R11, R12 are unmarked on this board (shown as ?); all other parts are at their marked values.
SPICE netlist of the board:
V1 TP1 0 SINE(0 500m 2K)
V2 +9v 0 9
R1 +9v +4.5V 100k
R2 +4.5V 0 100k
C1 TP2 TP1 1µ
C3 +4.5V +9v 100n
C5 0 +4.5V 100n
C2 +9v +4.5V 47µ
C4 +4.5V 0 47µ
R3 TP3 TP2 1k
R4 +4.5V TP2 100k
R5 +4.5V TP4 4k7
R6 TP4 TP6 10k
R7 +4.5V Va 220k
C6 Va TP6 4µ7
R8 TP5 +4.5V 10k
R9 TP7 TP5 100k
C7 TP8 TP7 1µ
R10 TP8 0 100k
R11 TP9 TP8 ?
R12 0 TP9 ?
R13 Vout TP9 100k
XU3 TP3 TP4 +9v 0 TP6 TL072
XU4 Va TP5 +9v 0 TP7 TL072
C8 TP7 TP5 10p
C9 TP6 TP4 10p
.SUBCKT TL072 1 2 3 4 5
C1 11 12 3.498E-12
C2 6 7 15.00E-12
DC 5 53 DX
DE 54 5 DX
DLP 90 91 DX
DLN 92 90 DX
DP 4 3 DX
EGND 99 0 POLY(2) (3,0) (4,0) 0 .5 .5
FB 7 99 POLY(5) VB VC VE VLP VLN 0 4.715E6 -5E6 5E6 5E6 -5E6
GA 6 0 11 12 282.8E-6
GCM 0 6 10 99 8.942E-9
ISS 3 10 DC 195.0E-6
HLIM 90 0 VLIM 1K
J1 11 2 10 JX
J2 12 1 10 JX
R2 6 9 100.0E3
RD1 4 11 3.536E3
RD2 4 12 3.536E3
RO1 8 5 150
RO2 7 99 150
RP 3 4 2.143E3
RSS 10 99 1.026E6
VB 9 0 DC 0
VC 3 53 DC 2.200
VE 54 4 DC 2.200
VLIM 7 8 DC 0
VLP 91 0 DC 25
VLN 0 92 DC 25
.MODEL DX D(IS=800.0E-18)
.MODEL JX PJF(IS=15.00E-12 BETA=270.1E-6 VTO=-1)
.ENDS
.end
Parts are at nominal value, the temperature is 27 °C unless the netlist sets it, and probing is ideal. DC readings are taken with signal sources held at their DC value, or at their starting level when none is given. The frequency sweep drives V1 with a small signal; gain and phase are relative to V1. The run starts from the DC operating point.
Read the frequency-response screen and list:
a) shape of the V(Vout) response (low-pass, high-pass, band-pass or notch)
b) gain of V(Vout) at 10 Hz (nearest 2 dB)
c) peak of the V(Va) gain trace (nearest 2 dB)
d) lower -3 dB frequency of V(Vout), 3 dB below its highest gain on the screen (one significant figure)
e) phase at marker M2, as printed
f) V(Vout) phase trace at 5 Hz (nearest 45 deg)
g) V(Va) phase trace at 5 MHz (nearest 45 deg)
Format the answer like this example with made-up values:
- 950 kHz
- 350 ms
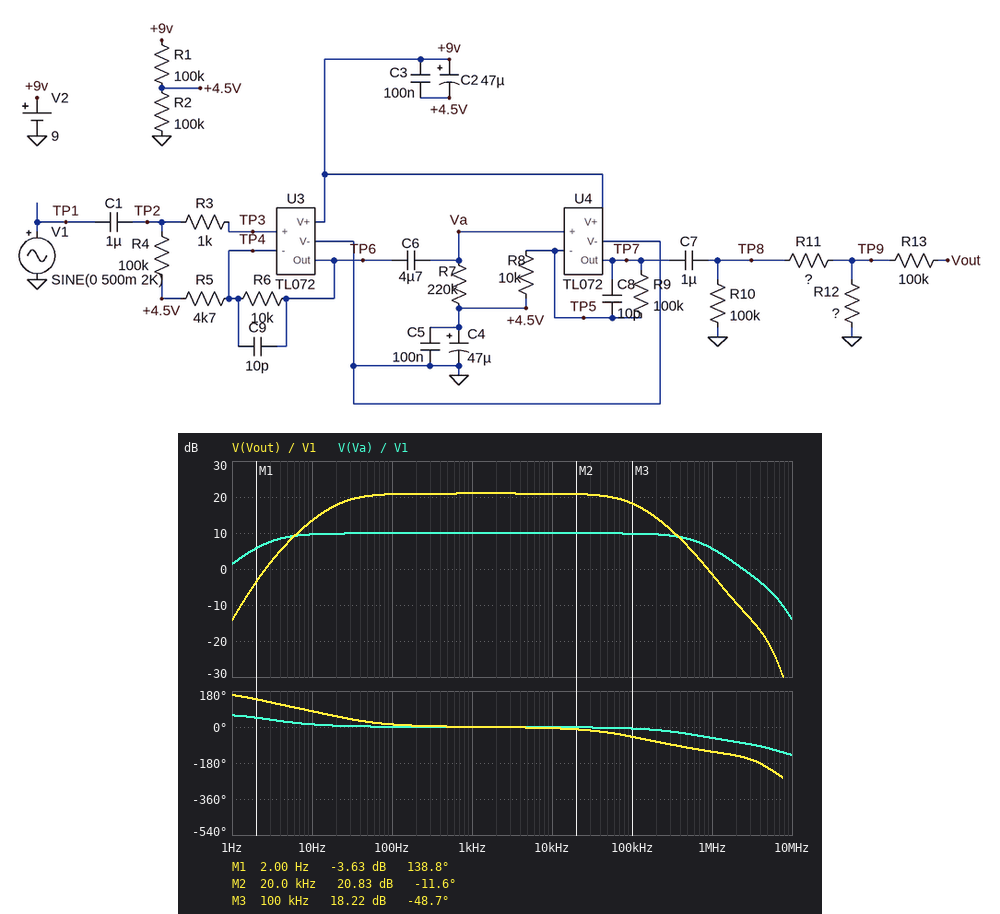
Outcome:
- band-pass
- 14 dB
- 10 dB
- 20 Hz
- -11.6 deg
- 90 deg
- -90 deg
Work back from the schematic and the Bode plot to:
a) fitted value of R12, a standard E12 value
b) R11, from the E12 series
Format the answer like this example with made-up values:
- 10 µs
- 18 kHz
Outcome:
- 2.7 kΩ
- 5.6 kΩ
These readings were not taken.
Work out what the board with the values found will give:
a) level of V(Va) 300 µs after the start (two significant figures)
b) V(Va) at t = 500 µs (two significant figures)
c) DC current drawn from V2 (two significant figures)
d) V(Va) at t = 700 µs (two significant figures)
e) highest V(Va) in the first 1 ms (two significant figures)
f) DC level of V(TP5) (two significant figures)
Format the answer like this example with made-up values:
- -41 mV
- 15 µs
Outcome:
- 3.6 V
- 4.5 V
- 8.8 mA
- 5.4 V
- 6.1 V
- 4.5 V
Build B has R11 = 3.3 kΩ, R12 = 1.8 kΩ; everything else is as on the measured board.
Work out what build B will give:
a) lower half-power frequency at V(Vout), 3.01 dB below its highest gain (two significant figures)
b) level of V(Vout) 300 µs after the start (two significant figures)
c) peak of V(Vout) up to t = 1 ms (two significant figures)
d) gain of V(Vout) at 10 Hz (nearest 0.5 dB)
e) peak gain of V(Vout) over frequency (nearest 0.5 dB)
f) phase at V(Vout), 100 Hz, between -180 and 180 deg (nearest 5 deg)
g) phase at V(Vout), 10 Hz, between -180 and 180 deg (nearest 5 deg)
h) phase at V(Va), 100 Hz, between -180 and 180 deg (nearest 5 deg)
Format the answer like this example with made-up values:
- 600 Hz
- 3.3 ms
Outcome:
- 33 Hz
- -1.1 V
- 1.0 V
- 10.5 dB
- 21.5 dB
- 20 deg
- 90 deg
- 0 deg
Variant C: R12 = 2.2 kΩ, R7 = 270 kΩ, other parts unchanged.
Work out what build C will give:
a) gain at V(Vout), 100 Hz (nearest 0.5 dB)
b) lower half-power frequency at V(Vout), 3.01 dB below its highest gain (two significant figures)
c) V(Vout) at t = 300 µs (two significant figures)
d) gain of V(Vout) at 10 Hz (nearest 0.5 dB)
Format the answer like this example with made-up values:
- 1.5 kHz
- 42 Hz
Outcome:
- 19.5 dB
- 22 Hz
- -860 mV
- 12.0 dB
